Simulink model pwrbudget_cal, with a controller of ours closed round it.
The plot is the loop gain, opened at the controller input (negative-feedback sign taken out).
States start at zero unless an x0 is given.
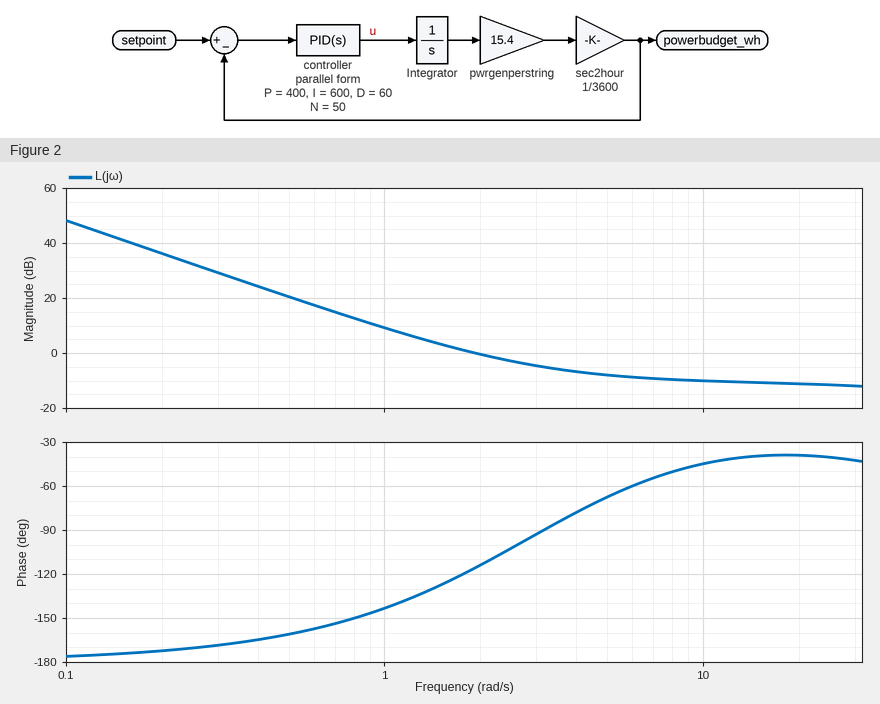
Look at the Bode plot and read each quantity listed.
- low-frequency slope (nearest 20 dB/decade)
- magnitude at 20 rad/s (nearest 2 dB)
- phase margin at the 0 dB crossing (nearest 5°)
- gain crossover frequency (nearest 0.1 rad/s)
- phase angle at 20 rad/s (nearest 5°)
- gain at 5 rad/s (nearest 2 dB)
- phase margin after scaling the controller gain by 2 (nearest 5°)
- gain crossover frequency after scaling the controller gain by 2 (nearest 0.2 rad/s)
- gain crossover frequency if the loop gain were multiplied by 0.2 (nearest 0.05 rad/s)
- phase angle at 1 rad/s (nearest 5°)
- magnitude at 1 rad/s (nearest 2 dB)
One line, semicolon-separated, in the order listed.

-40 dB/decade; -12 dB; 65°; 1.9 rad/s; -40°; -8 dB; 95°; 3.6 rad/s; 0.75 rad/s; -145°; 10 dB
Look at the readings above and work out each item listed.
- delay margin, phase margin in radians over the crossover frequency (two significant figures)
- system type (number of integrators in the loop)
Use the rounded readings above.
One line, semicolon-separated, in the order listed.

0.60 s; 2
